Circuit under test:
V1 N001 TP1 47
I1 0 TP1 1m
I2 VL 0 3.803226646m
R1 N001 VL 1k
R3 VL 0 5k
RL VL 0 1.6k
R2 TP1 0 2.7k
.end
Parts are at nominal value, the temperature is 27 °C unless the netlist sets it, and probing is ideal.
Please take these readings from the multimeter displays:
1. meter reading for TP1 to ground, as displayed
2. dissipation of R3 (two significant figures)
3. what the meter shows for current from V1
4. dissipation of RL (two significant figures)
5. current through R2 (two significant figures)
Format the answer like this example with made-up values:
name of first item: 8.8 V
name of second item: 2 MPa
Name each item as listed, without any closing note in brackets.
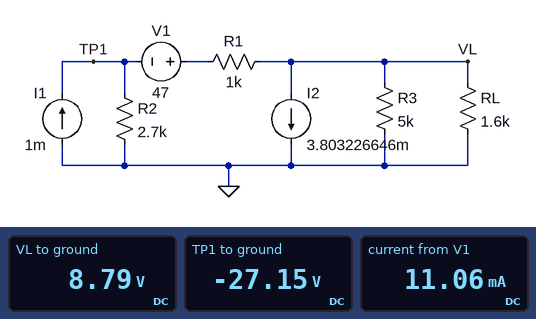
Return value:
meter reading for TP1 to ground, as displayed: -27.15 V
dissipation of R3: 15 mW
what the meter shows for current from V1: 11.06 mA
dissipation of RL: 48 mW
current through R2: 10 mA
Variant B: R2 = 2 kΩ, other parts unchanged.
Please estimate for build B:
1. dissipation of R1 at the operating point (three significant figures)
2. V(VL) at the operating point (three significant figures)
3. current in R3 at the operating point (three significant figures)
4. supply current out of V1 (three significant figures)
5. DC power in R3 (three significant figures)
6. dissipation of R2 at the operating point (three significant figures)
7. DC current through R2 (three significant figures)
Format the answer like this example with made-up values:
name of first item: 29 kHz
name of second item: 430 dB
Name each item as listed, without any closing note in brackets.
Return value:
dissipation of R1 at the operating point: 162 mW
V(VL) at the operating point: 10.8 V
current in R3 at the operating point: 2.16 mA
supply current out of V1: 12.7 mA
DC power in R3: 23.4 mW
dissipation of R2 at the operating point: 275 mW
DC current through R2: 11.7 mA
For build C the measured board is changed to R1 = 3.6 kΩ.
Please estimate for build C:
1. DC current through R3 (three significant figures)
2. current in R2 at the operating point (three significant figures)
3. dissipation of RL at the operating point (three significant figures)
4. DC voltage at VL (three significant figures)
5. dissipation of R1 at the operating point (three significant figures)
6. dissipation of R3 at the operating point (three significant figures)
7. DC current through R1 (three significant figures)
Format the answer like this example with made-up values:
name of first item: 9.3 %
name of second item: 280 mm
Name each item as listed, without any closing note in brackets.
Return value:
DC current through R3: 831 µA
current in R2 at the operating point: 6.23 mA
dissipation of RL at the operating point: 10.8 mW
DC voltage at VL: 4.15 V
dissipation of R1 at the operating point: 188 mW
dissipation of R3 at the operating point: 3.45 mW
DC current through R1: 7.23 mA
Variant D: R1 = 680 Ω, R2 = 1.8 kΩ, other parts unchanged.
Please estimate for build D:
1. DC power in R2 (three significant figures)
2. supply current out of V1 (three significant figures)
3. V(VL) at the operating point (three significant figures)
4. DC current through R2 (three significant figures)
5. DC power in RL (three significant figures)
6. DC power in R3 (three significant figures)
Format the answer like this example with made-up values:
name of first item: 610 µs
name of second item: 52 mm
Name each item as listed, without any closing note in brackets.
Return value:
DC power in R2: 326 mW
supply current out of V1: 14.5 mA
V(VL) at the operating point: 12.9 V
DC current through R2: 13.5 mA
DC power in RL: 104 mW
DC power in R3: 33.4 mW
